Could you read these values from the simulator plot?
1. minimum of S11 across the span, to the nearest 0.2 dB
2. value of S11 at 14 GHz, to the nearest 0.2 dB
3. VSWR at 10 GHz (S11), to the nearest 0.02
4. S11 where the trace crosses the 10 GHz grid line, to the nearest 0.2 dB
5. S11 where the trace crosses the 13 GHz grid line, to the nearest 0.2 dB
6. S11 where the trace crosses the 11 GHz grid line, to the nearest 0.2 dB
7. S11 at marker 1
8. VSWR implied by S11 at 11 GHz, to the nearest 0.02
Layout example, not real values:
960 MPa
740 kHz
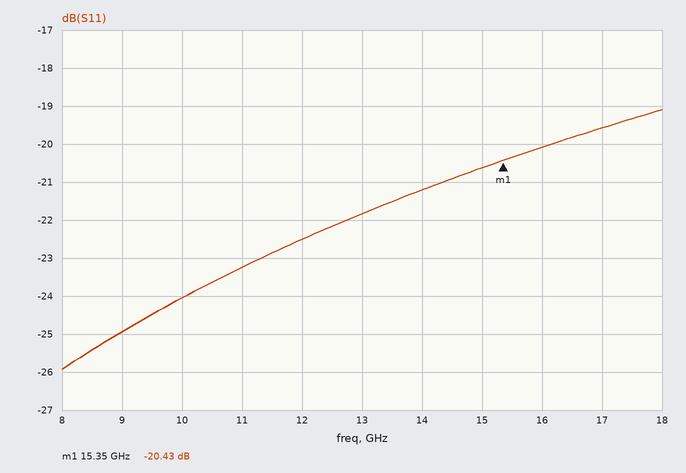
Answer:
-26.0 dB
-21.2 dB
1.14
-24.0 dB
-21.8 dB
-23.2 dB
-20.43 dB
1.14
